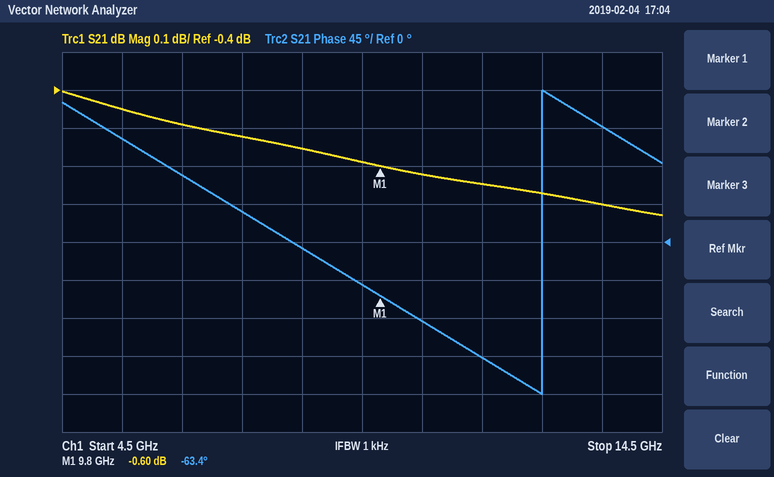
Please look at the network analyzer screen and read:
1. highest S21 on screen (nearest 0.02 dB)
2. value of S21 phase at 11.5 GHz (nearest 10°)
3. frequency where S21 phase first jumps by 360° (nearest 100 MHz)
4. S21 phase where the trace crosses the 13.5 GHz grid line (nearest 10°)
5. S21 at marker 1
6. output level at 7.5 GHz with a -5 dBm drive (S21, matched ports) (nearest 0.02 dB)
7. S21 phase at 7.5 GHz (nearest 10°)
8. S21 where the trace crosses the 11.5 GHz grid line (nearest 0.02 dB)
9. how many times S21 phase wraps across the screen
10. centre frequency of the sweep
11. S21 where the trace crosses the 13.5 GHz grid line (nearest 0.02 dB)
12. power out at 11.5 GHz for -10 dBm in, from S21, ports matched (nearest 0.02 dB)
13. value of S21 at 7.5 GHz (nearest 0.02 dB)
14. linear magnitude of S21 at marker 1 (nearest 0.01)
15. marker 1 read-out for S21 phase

-0.40 dB
-140°
12.5 GHz
140°
-0.60 dB
-5.52 dBm
40°
-0.64 dB
1
9.5 GHz
-0.70 dB
-10.64 dBm
-0.52 dB
0.93
-63.4°
